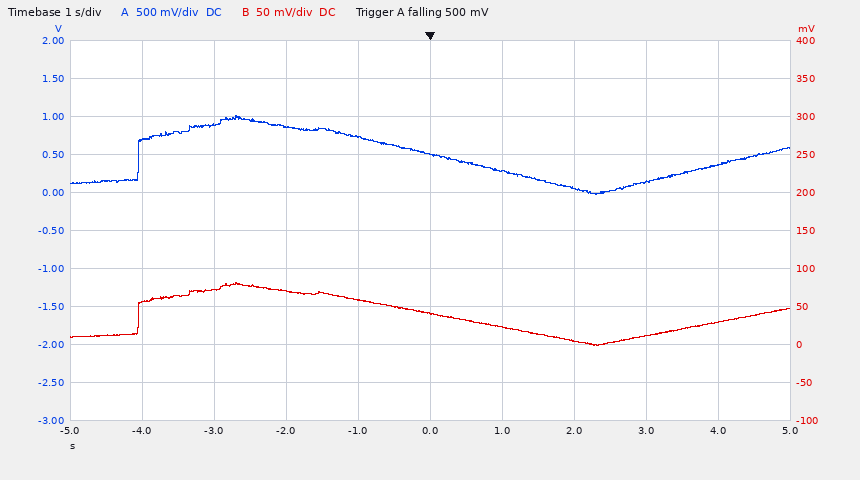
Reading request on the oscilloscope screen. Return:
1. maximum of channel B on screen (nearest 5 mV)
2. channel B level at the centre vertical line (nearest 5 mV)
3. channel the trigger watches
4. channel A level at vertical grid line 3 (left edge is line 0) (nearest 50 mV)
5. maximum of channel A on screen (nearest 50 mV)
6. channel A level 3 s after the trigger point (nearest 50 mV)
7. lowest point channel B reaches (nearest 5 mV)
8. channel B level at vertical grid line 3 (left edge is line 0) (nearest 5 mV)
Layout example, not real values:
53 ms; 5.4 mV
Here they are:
80 mV; 40 mV; channel A; 850 mV; 1.00 V; 150 mV; 0 mV; 70 mV
